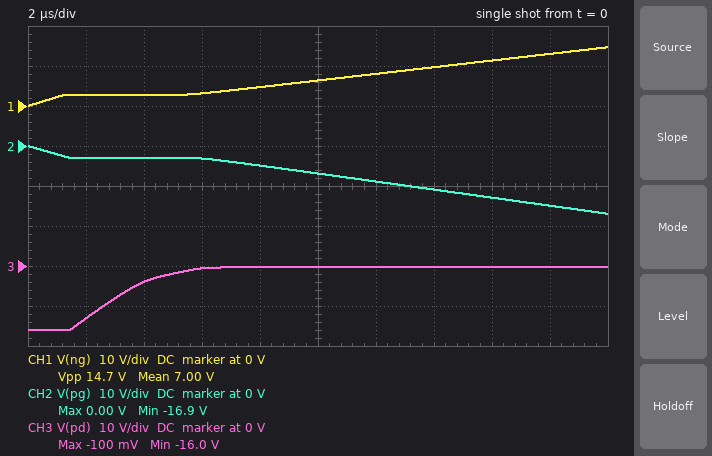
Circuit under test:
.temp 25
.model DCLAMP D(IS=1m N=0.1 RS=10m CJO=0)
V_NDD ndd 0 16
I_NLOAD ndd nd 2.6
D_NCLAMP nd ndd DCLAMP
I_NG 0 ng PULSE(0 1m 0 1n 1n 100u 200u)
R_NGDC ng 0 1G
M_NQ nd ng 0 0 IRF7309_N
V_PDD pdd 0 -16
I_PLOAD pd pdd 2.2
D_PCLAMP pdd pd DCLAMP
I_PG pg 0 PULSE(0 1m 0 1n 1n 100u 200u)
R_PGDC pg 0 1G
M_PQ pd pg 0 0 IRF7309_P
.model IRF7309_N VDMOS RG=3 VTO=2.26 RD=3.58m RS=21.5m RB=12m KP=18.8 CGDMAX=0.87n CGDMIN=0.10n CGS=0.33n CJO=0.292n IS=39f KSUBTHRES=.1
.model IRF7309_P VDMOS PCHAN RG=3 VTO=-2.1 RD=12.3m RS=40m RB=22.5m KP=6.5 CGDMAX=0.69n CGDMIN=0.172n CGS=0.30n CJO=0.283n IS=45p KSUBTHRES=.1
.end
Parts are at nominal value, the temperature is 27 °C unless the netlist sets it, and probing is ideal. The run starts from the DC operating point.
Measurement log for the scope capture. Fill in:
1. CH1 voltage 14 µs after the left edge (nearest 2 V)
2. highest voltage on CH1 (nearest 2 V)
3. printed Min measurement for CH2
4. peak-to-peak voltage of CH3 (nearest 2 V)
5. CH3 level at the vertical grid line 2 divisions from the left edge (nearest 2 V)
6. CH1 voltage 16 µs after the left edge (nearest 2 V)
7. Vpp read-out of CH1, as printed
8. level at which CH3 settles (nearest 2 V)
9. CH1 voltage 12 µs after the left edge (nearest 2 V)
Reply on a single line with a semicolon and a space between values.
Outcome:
10 V; 14 V; -16.9 V; 16 V; -4 V; 12 V; 14.7 V; 0 V; 8 V
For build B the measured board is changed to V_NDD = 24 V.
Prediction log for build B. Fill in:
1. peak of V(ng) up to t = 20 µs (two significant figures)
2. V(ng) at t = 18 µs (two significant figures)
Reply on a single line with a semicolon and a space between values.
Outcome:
14 V; 12 V
